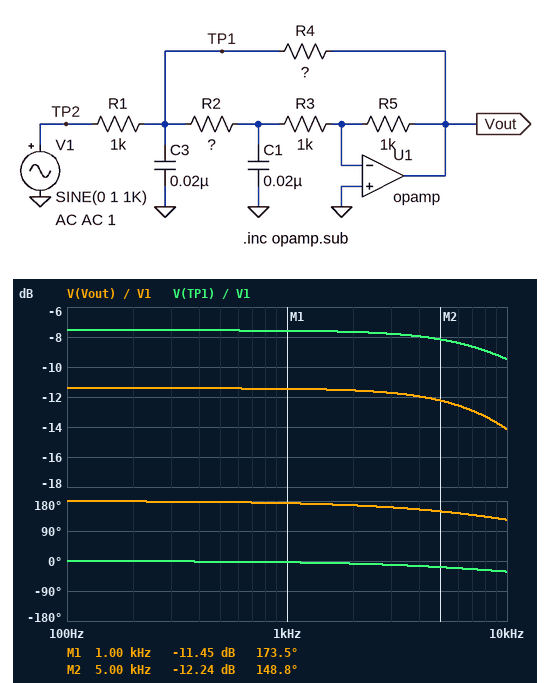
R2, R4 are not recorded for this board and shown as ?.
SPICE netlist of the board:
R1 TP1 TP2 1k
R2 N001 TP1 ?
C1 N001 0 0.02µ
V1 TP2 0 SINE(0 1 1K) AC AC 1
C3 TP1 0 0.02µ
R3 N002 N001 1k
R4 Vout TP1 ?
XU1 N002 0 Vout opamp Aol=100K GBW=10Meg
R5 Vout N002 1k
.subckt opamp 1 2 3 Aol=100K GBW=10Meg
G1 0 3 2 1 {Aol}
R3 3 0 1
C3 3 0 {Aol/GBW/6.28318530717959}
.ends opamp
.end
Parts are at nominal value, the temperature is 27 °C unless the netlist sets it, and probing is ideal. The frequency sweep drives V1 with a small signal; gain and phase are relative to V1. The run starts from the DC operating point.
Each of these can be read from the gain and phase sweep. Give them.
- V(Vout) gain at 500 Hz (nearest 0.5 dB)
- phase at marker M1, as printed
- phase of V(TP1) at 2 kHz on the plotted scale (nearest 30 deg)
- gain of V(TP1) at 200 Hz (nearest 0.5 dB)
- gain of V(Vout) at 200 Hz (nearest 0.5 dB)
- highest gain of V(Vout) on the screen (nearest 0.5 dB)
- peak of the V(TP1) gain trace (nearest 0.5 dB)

-11.5 dB
173.5 deg
0 deg
-7.5 dB
-11.5 dB
-11.5 dB
-7.5 dB
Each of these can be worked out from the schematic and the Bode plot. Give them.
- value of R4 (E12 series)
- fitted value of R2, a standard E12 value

2.2 kΩ
560 Ω
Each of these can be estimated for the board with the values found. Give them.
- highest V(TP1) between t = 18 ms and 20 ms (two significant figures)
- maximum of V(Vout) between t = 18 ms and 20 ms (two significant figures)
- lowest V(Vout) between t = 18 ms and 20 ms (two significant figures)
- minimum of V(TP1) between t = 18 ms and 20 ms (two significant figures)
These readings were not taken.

420 mV
270 mV
-270 mV
-420 mV
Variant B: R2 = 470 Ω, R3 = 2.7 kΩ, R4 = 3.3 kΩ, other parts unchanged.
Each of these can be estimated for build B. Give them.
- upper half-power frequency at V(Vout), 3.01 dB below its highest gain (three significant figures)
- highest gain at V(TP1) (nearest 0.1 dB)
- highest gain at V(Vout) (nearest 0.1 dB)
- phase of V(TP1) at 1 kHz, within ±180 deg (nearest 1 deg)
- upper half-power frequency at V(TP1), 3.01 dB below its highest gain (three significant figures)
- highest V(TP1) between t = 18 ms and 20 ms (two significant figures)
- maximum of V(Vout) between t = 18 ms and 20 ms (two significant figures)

6.53 kHz
-4.7 dB
-14.7 dB
-7 deg
7.34 kHz
580 mV
180 mV
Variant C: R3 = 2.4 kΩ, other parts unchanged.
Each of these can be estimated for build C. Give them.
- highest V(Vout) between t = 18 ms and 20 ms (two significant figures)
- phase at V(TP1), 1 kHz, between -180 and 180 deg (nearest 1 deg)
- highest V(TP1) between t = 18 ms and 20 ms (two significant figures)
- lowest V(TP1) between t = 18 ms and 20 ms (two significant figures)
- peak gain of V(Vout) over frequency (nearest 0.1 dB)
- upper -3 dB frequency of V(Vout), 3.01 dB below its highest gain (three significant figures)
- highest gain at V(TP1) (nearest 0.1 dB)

170 mV
-6 deg
510 mV
-510 mV
-15.2 dB
7.29 kHz
-5.8 dB
